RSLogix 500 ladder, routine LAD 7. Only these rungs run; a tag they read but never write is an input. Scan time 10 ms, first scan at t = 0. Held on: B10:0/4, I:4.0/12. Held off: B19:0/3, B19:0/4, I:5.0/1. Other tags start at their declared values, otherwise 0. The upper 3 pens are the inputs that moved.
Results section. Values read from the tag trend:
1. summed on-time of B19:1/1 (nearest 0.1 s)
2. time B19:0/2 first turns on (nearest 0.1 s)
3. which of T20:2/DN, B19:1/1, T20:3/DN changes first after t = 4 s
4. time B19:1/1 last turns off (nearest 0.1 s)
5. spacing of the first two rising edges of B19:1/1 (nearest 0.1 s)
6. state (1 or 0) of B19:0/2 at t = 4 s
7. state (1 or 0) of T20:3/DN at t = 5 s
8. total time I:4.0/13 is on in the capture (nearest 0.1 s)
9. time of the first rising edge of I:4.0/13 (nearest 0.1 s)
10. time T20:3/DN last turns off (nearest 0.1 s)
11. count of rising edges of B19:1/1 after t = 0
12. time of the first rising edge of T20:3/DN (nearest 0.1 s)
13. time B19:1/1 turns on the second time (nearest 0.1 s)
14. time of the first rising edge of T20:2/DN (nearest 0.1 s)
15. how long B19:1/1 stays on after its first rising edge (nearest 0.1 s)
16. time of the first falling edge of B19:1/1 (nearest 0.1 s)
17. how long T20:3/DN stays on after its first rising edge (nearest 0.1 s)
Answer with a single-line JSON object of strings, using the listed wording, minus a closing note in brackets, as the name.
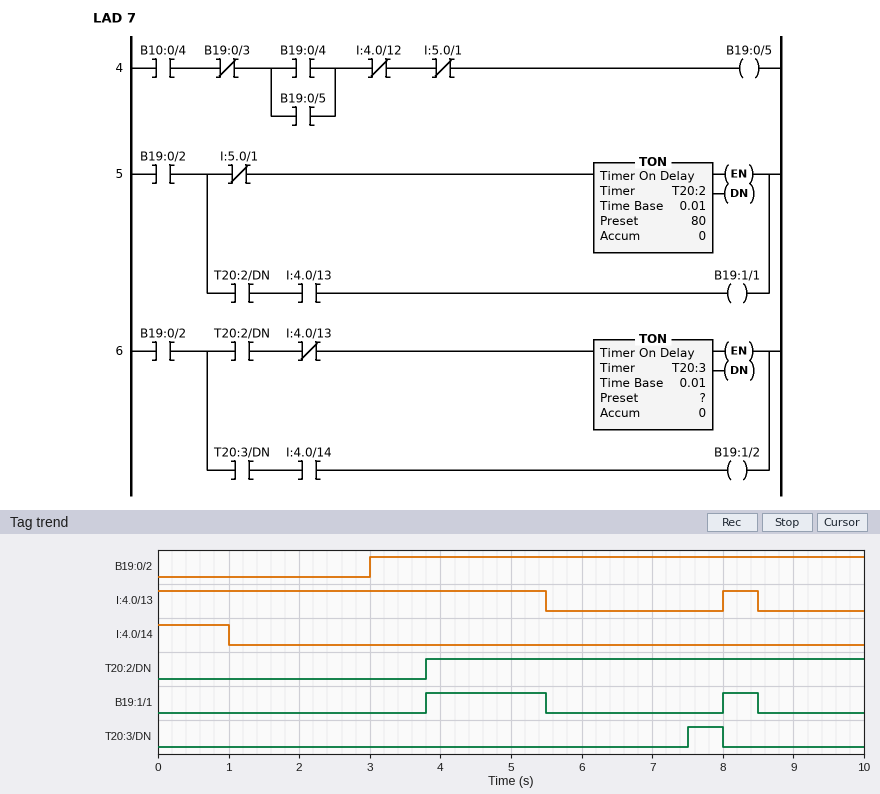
{"summed on-time of B19:1/1": "2.2 s", "time B19:0/2 first turns on": "3.0 s", "which of T20:2/DN, B19:1/1, T20:3/DN changes first after t = 4 s": "B19:1/1", "time B19:1/1 last turns off": "8.5 s", "spacing of the first two rising edges of B19:1/1": "4.2 s", "state (1 or 0) of B19:0/2 at t = 4 s": "1", "state (1 or 0) of T20:3/DN at t = 5 s": "0", "total time I:4.0/13 is on in the capture": "6.0 s", "time of the first rising edge of I:4.0/13": "8.0 s", "time T20:3/DN last turns off": "8.0 s", "count of rising edges of B19:1/1 after t = 0": "2", "time of the first rising edge of T20:3/DN": "7.5 s", "time B19:1/1 turns on the second time": "8.0 s", "time of the first rising edge of T20:2/DN": "3.8 s", "how long B19:1/1 stays on after its first rising edge": "1.7 s", "time of the first falling edge of B19:1/1": "5.5 s", "how long T20:3/DN stays on after its first rising edge": "0.5 s"}
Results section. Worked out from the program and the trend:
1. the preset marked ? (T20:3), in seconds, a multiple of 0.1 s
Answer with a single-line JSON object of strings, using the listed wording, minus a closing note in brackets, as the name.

{"the preset marked ? (T20:3), in seconds, a multiple of 0.1 s": "2.0 s"}
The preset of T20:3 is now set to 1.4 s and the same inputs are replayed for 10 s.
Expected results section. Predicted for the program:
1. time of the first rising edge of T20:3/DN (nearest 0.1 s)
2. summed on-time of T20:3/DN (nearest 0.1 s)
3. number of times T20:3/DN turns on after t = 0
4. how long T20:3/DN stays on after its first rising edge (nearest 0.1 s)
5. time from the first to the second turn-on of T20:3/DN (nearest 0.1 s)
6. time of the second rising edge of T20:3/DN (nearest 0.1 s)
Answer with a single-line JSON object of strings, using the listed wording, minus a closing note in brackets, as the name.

{"time of the first rising edge of T20:3/DN": "6.9 s", "summed on-time of T20:3/DN": "1.2 s", "number of times T20:3/DN turns on after t = 0": "2", "how long T20:3/DN stays on after its first rising edge": "1.1 s", "time from the first to the second turn-on of T20:3/DN": "3.0 s", "time of the second rising edge of T20:3/DN": "9.9 s"}
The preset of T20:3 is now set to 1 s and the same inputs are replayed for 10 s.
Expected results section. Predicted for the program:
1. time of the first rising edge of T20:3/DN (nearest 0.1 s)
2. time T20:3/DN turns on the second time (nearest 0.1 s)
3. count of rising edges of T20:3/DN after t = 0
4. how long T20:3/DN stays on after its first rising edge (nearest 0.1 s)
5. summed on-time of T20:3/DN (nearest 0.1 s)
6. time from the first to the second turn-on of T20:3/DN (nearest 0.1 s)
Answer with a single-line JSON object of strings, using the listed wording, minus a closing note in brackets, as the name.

{"time of the first rising edge of T20:3/DN": "6.5 s", "time T20:3/DN turns on the second time": "9.5 s", "count of rising edges of T20:3/DN after t = 0": "2", "how long T20:3/DN stays on after its first rising edge": "1.5 s", "summed on-time of T20:3/DN": "2.0 s", "time from the first to the second turn-on of T20:3/DN": "3.0 s"}
